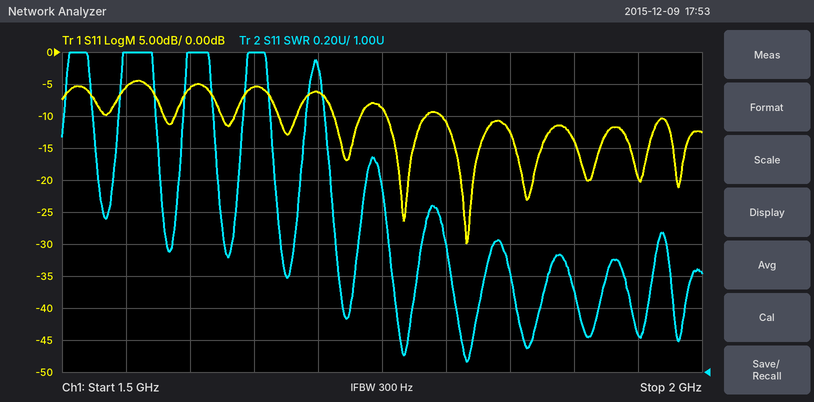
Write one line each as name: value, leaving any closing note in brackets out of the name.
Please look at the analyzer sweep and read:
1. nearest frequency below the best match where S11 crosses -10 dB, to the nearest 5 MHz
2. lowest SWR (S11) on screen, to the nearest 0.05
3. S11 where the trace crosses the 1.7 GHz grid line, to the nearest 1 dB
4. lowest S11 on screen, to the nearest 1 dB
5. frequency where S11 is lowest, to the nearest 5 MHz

nearest frequency below the best match where S11 crosses -10 dB, to the nearest 5 MHz: 1.795 GHz
lowest SWR (S11) on screen, to the nearest 0.05: 1.05
S11 where the trace crosses the 1.7 GHz grid line, to the nearest 1 dB: -6 dB
lowest S11 on screen, to the nearest 1 dB: -30 dB
frequency where S11 is lowest, to the nearest 5 MHz: 1.815 GHz
